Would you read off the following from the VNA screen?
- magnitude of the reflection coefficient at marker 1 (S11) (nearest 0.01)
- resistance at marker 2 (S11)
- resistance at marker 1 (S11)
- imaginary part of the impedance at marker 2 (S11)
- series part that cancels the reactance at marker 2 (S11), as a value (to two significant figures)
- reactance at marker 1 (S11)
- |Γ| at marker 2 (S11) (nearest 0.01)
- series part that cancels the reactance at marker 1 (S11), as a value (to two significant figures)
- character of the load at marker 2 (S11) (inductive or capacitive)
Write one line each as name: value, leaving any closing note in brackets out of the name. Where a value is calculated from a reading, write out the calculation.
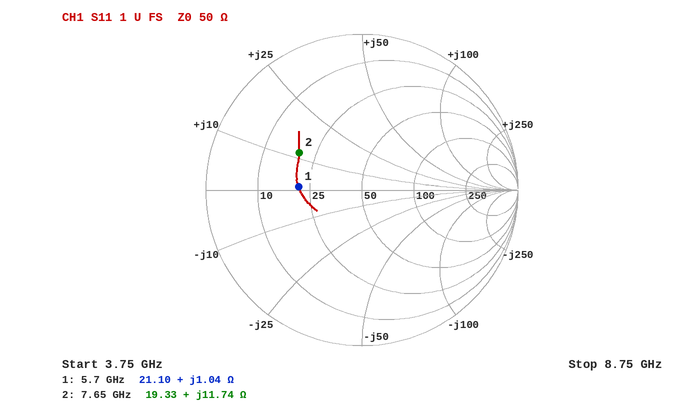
magnitude of the reflection coefficient at marker 1 (S11): 0.41
resistance at marker 2: 19.33 Ω
resistance at marker 1: 21.10 Ω
imaginary part of the impedance at marker 2: +11.74 Ω
series part that cancels the reactance at marker 2 (S11), as a value: C = 1/(2π × 7.65 GHz × 11.74 Ω) ≈ 1.8 pF
reactance at marker 1: +1.04 Ω
|Γ| at marker 2 (S11): 0.47
series part that cancels the reactance at marker 1 (S11), as a value: C = 1/(2π × 5.7 GHz × 1.04 Ω) ≈ 27 pF
character of the load at marker 2 (S11): inductive
